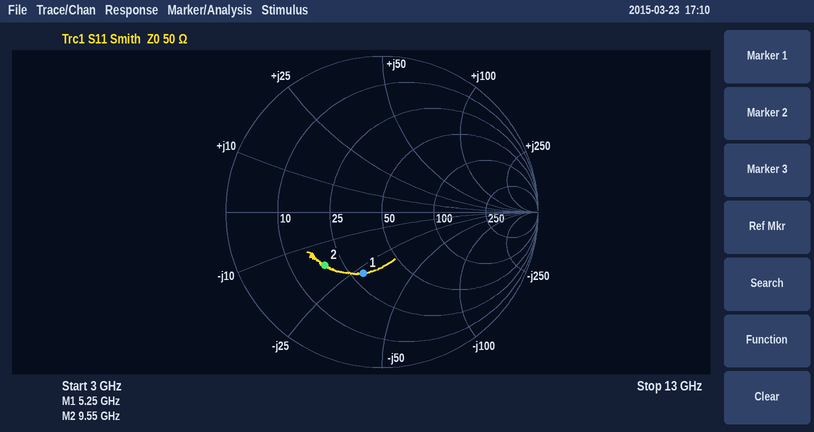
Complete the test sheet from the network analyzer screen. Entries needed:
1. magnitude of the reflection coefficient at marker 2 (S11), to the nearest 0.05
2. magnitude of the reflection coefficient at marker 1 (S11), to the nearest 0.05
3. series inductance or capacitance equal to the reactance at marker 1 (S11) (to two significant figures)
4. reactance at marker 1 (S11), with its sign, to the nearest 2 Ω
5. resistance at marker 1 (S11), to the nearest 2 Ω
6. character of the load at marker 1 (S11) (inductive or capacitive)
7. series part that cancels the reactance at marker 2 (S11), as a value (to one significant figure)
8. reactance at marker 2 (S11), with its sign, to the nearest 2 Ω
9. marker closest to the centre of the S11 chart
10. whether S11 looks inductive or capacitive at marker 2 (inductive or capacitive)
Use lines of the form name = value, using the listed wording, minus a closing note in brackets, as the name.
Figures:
magnitude of the reflection coefficient at marker 2 (S11), to the nearest 0.05 = 0.50
magnitude of the reflection coefficient at marker 1 (S11), to the nearest 0.05 = 0.40
series inductance or capacitance equal to the reactance at marker 1 (S11) = 1.1 pF
reactance at marker 1 (S11), with its sign, to the nearest 2 Ω = -28 Ω
resistance at marker 1 (S11), to the nearest 2 Ω = 30 Ω
character of the load at marker 1 (S11) = capacitive
series part that cancels the reactance at marker 2 (S11), as a value = 300 pH
reactance at marker 2 (S11), with its sign, to the nearest 2 Ω = -18 Ω
marker closest to the centre of the S11 chart = marker 1
whether S11 looks inductive or capacitive at marker 2 = capacitive
